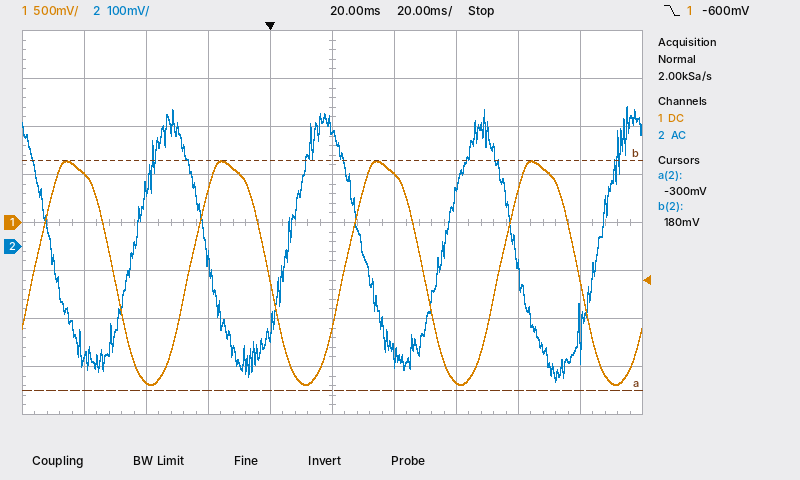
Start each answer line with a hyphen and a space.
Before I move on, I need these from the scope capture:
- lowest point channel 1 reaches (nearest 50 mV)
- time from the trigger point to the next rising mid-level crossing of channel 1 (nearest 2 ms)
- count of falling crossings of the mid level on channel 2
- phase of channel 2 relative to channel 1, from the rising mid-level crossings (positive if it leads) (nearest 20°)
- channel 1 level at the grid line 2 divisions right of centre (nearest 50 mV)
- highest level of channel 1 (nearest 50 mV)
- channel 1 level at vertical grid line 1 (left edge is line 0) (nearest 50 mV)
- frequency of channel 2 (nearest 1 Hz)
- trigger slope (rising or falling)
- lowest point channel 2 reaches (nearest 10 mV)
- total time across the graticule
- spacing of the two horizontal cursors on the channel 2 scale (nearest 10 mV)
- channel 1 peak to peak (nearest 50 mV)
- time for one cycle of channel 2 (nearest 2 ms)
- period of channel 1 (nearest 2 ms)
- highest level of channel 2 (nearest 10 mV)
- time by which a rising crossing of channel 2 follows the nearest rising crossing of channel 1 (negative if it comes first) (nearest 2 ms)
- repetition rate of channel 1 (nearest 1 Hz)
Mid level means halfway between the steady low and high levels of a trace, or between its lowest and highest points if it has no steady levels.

- -1.70 V
- 24 ms
- 4
- +120°
- -1.65 V
- 650 mV
- 500 mV
- 20 Hz
- falling
- -280 mV
- 200 ms
- 480 mV
- 2.35 V
- 50 ms
- 50 ms
- 290 mV
- -18 ms
- 20 Hz
